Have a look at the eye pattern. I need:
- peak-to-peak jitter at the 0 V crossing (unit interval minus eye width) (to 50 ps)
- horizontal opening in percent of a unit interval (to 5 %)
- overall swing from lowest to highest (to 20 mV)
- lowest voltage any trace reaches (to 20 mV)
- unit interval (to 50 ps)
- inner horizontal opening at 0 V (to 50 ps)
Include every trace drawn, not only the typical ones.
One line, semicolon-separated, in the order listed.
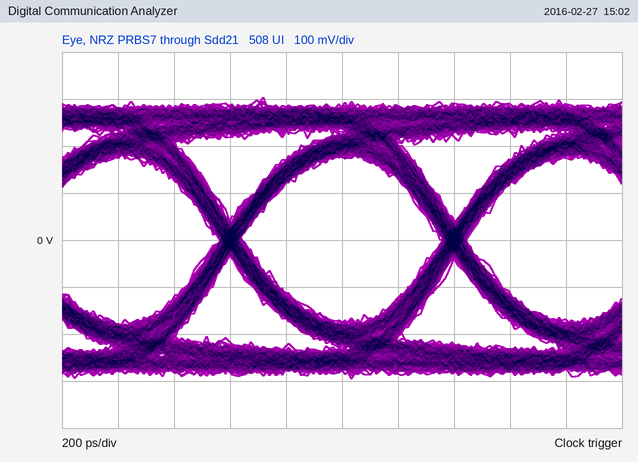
100 ps; 90 %; 600 mV; -300 mV; 800 ps; 700 ps
